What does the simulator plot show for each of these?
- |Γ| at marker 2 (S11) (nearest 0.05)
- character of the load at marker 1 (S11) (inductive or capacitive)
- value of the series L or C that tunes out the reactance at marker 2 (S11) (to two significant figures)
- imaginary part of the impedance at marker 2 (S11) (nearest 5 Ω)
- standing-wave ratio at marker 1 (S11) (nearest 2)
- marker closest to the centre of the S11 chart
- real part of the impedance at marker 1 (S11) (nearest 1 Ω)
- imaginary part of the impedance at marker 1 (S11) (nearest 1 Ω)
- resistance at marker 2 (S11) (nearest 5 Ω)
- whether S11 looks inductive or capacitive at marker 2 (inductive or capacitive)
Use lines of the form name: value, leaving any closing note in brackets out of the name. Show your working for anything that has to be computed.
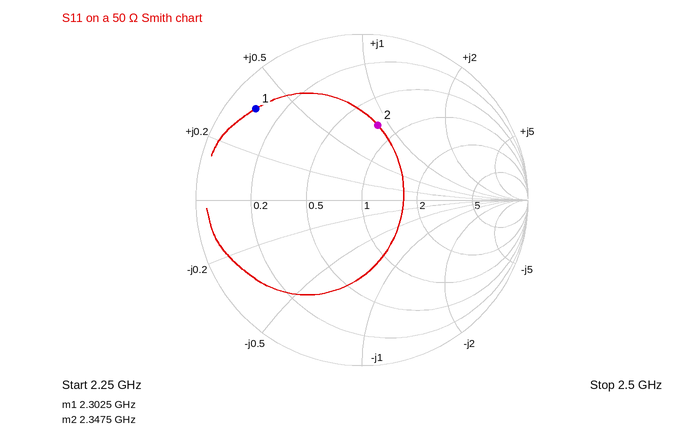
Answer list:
|Γ| at marker 2 (S11): 0.45
character of the load at marker 1 (S11): inductive
value of the series L or C that tunes out the reactance at marker 2 (S11): C = 1/(2π × 2.3475 GHz × 45 Ω) ≈ 1.5 pF
imaginary part of the impedance at marker 2 (S11): +45 Ω
standing-wave ratio at marker 1 (S11): 12
marker closest to the centre of the S11 chart: marker 2
real part of the impedance at marker 1 (S11): 5 Ω
imaginary part of the impedance at marker 1 (S11): +18 Ω
resistance at marker 2 (S11): 40 Ω
whether S11 looks inductive or capacitive at marker 2: inductive
